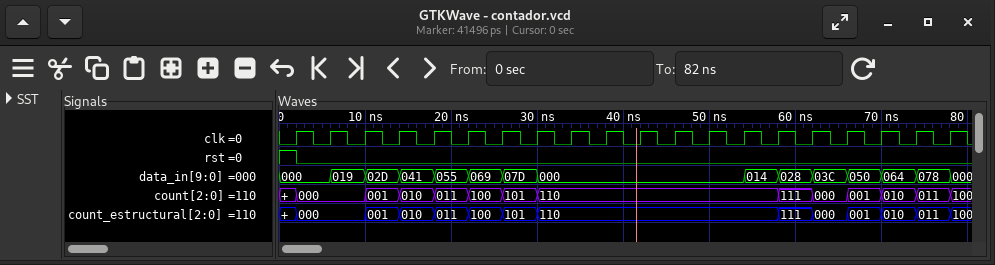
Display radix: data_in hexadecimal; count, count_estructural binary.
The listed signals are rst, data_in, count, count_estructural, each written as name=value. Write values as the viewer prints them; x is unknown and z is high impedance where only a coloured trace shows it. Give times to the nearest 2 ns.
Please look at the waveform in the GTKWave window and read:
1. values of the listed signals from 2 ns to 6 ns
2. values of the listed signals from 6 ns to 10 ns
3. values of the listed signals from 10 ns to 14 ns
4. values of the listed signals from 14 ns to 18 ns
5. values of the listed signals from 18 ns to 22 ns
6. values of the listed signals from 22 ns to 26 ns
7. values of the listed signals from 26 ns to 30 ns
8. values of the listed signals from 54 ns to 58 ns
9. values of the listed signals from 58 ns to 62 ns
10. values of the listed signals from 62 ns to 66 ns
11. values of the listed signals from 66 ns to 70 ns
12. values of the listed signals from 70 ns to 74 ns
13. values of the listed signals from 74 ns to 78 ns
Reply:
rst=0, data_in=000, count=000, count_estructural=000
rst=0, data_in=019, count=000, count_estructural=000
rst=0, data_in=02D, count=001, count_estructural=001
rst=0, data_in=041, count=010, count_estructural=010
rst=0, data_in=055, count=011, count_estructural=011
rst=0, data_in=069, count=100, count_estructural=100
rst=0, data_in=07D, count=101, count_estructural=101
rst=0, data_in=014, count=110, count_estructural=110
rst=0, data_in=028, count=111, count_estructural=111
rst=0, data_in=03C, count=000, count_estructural=000
rst=0, data_in=050, count=001, count_estructural=001
rst=0, data_in=064, count=010, count_estructural=010
rst=0, data_in=078, count=011, count_estructural=011
